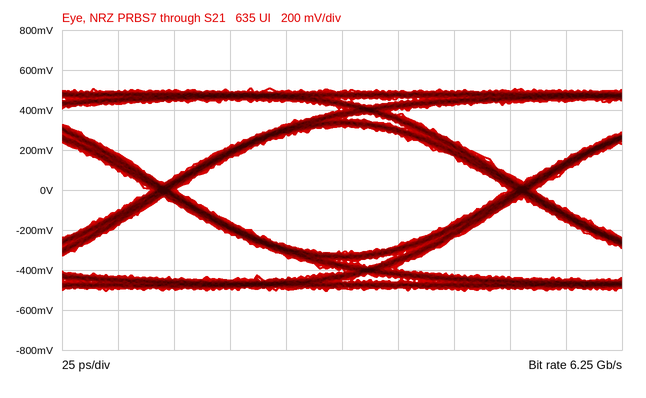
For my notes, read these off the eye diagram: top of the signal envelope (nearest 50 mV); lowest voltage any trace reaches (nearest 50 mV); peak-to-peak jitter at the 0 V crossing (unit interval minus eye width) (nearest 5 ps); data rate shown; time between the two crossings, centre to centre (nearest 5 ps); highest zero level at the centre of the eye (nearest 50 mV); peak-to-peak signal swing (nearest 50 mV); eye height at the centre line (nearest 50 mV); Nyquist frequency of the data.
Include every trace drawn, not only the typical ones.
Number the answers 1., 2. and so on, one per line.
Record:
1. 500 mV
2. -500 mV
3. 10 ps
4. 6.25 Gb/s
5. 160 ps
6. -300 mV
7. 1.00 V
8. 650 mV
9. 3.125 GHz
